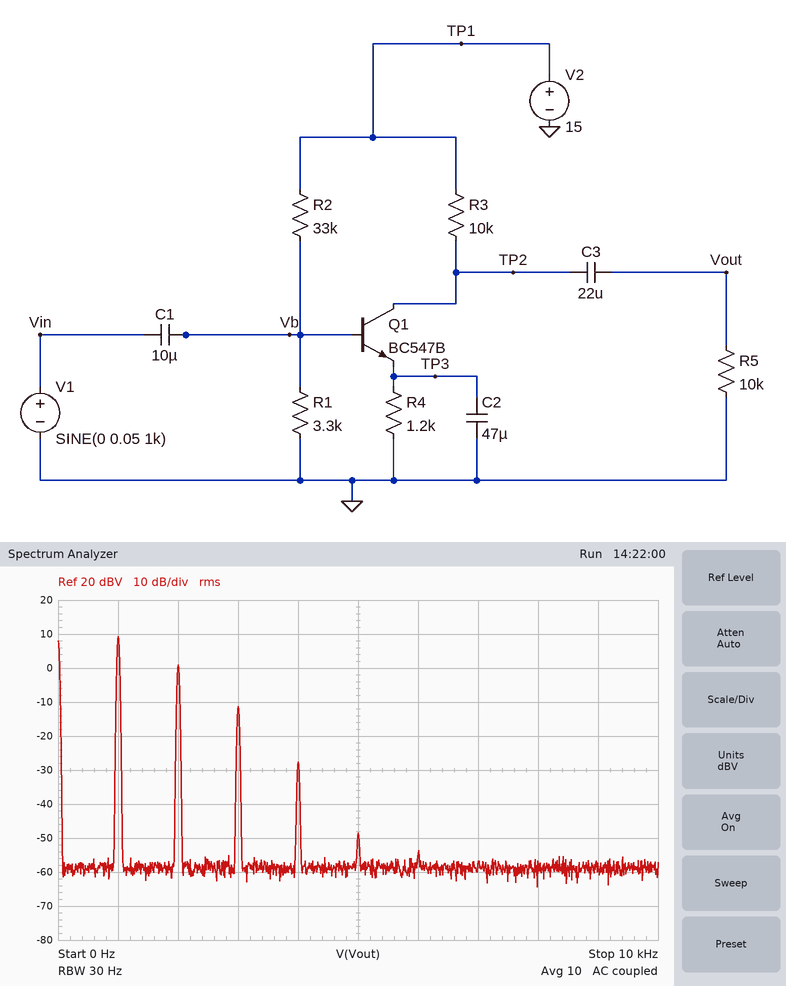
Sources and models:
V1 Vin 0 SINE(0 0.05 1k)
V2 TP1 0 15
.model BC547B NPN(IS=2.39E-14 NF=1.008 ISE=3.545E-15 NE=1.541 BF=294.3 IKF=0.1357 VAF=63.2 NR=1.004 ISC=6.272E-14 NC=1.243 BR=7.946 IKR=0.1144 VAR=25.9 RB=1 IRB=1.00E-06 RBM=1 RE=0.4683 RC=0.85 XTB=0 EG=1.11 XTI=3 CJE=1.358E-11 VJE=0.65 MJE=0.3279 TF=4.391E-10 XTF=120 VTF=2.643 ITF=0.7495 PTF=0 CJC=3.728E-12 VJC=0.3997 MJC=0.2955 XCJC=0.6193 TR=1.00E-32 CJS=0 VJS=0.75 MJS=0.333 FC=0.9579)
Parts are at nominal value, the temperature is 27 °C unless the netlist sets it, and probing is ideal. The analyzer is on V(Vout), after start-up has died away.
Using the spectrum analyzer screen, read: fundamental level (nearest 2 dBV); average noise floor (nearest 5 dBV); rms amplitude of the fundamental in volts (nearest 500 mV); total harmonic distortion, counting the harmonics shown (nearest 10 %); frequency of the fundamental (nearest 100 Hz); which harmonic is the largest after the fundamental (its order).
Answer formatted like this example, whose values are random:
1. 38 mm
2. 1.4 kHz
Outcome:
1. 10 dBV
2. -60 dBV
3. 3.0 V
4. 40 %
5. 1.0 kHz
6. 2
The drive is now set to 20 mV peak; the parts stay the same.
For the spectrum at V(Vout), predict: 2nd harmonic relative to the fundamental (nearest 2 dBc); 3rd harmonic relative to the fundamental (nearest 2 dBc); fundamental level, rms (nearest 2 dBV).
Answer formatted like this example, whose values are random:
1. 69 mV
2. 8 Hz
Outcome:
1. -16 dBc
2. -36 dBc
3. 4 dBV
